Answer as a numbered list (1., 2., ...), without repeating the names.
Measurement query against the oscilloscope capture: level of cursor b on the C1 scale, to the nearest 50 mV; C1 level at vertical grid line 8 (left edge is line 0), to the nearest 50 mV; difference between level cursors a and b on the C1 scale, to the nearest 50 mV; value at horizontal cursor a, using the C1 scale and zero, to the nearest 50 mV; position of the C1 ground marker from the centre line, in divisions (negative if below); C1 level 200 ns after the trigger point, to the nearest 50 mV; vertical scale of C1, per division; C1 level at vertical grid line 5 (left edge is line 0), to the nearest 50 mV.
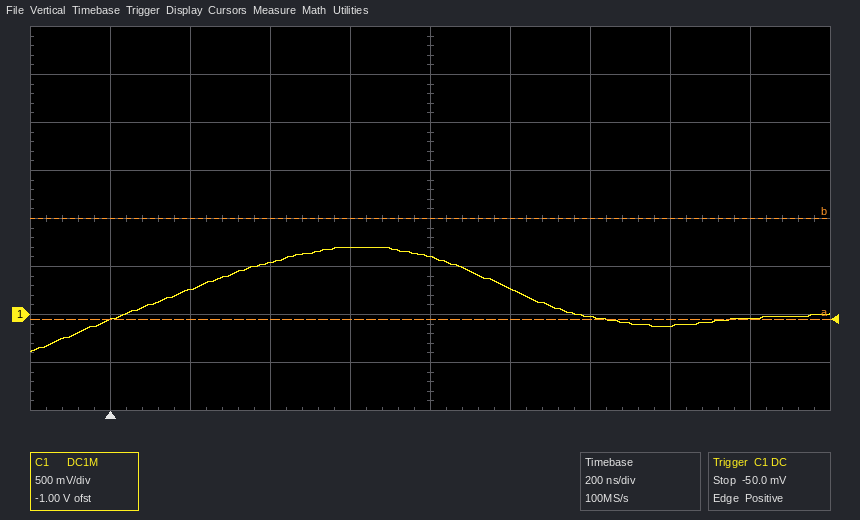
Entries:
1. 1.00 V
2. -100 mV
3. 1.05 V
4. -50 mV
5. -2.0 div
6. 250 mV
7. 500 mV
8. 600 mV
